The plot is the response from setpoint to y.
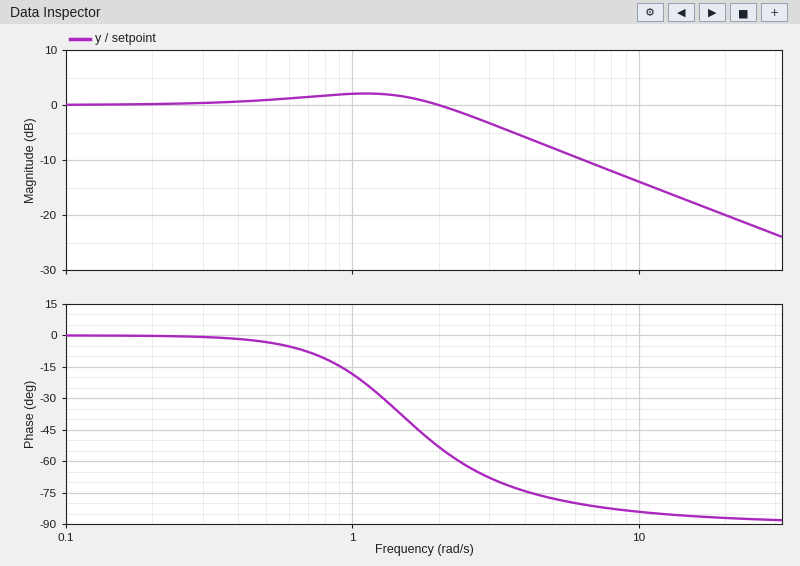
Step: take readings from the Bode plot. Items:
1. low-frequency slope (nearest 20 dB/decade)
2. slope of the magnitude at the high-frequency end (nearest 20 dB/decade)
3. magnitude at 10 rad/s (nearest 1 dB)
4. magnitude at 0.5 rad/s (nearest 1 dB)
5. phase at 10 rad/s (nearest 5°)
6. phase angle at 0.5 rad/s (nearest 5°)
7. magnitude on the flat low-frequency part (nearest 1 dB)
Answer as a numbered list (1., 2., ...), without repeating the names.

1. 0 dB/decade
2. -20 dB/decade
3. -14 dB
4. 1 dB
5. -85°
6. -5°
7. 0 dB
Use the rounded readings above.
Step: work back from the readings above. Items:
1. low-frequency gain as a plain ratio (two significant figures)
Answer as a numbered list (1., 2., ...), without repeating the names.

1. 1.0
